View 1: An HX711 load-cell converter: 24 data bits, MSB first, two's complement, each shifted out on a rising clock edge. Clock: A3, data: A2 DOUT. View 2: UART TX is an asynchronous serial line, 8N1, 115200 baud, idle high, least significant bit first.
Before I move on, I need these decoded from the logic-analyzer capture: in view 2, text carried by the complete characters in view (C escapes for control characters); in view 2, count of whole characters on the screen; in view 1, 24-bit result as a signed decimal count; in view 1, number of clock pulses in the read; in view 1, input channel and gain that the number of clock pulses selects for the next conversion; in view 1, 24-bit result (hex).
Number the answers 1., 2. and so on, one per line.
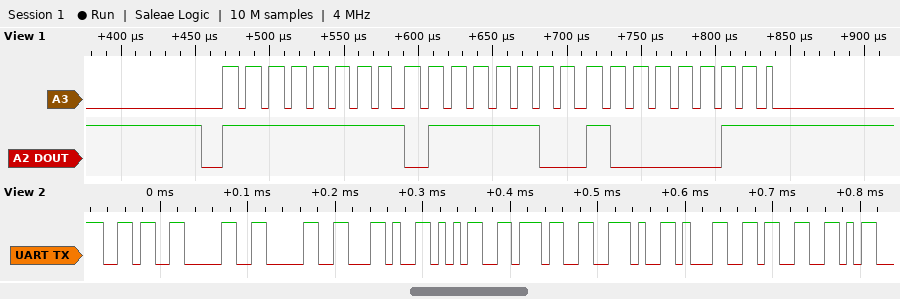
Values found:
1. "600,57.13"
2. 9
3. -33661
4. 25
5. channel A, gain 128
6. 0xFF7C83
